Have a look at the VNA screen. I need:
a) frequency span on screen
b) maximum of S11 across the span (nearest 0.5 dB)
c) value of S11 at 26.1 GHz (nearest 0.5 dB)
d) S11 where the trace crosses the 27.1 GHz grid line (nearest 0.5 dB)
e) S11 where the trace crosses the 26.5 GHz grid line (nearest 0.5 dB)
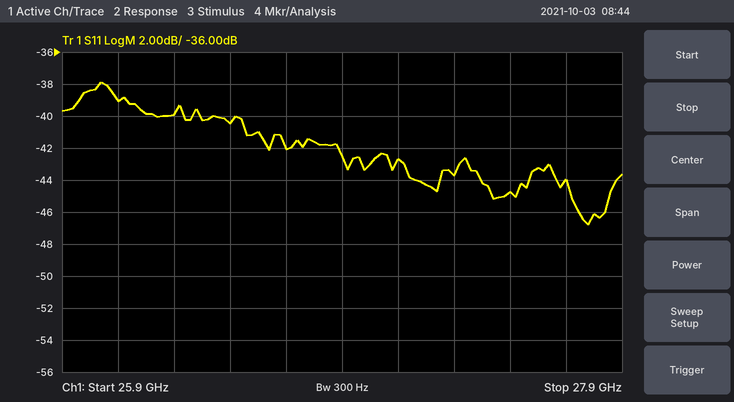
2 GHz
-38.0 dB
-39.0 dB
-42.5 dB
-40.5 dB
